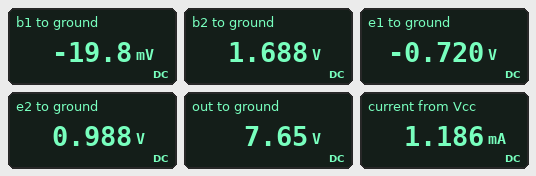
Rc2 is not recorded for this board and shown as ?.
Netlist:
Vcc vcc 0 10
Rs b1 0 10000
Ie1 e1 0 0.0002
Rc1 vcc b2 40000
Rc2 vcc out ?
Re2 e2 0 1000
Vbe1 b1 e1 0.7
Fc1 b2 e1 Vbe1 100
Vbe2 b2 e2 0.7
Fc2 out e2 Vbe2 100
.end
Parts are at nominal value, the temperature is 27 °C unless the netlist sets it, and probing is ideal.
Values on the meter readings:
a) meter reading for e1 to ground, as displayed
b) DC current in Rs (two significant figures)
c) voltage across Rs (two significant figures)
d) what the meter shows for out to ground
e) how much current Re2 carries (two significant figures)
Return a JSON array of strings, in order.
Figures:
["-0.720 V", "2.0 µA", "20 mV", "7.65 V", "990 µA"]
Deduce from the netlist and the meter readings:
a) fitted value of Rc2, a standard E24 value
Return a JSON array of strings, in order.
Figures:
["2.4 kΩ"]
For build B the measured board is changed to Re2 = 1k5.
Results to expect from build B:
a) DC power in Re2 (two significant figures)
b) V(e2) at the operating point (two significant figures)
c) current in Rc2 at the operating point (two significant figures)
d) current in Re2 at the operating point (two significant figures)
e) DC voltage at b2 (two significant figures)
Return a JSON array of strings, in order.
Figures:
["790 µW", "1.1 V", "720 µA", "730 µA", "1.8 V"]
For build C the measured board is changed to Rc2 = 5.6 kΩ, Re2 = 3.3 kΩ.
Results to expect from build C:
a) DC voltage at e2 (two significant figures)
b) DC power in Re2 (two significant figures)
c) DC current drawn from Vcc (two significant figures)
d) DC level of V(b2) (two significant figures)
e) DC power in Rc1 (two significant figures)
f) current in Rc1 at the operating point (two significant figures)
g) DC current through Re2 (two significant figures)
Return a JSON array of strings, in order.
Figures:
["1.2 V", "460 µW", "570 µA", "1.9 V", "1.6 mW", "200 µA", "370 µA"]
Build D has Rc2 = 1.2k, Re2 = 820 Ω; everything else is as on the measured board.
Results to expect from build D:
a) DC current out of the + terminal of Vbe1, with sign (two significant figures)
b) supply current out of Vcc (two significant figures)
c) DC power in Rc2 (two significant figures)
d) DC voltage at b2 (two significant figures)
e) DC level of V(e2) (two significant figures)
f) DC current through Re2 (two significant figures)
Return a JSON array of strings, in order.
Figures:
["-2.0 µA", "1.3 mA", "1.5 mW", "1.6 V", "930 mV", "1.1 mA"]
